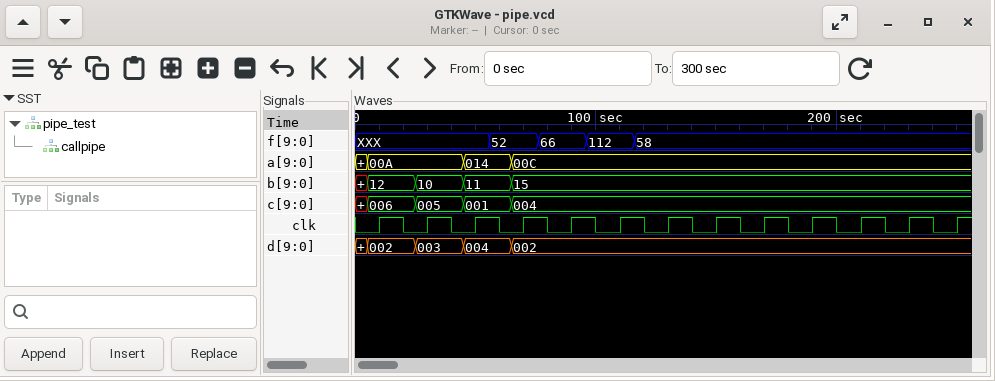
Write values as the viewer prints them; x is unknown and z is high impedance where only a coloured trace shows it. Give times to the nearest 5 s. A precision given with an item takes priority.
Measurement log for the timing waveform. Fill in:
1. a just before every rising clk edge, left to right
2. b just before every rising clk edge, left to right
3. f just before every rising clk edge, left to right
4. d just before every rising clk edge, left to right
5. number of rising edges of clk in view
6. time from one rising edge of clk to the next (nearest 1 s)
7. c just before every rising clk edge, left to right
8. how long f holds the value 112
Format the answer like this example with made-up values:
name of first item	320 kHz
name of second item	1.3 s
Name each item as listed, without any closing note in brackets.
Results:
a just before every rising clk edge, left to right	00A, 00A, 014, 00C, 00C, 00C, 00C, 00C, 00C, 00C, 00C, 00C, 00C
b just before every rising clk edge, left to right	12, 10, 11, 15, 15, 15, 15, 15, 15, 15, 15, 15, 15
f just before every rising clk edge, left to right	XXX, XXX, XXX, 52, 66, 112, 58, 58, 58, 58, 58, 58, 58
d just before every rising clk edge, left to right	002, 003, 004, 002, 002, 002, 002, 002, 002, 002, 002, 002, 002
number of rising edges of clk in view	13
time from one rising edge of clk to the next	20 s
c just before every rising clk edge, left to right	006, 005, 001, 004, 004, 004, 004, 004, 004, 004, 004, 004, 004
how long f holds the value 112	20 s
